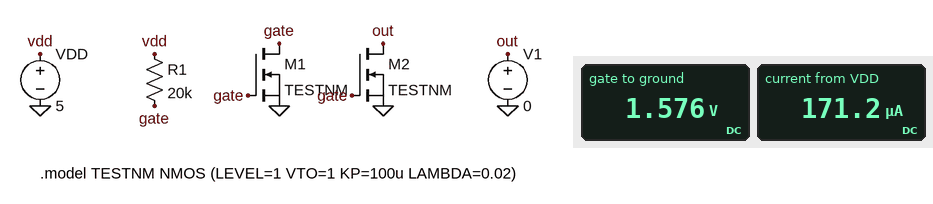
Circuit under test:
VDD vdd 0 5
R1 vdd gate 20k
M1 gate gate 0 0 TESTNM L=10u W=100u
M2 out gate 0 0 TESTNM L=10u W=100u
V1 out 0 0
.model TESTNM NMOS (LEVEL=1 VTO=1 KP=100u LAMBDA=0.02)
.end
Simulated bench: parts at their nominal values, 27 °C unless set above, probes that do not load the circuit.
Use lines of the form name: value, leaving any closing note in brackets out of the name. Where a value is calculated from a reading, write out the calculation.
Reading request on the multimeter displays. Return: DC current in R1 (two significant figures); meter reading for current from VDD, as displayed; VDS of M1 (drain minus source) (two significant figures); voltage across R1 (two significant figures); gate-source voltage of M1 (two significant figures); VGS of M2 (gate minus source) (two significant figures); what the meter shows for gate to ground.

DC current in R1: (5 V - 1.576 V) / 20 kΩ = 170 µA
meter reading for current from VDD, as displayed: 171.2 µA
VDS of M1 (drain minus source): 1.576 V = 1.6 V
voltage across R1: 5 V - 1.576 V = 3.4 V
gate-source voltage of M1: 1.576 V = 1.6 V
VGS of M2 (gate minus source): 1.576 V = 1.6 V
what the meter shows for gate to ground: 1.576 V
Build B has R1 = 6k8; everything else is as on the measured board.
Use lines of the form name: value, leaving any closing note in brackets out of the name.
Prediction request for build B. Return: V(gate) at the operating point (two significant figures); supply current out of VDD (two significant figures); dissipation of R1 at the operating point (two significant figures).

V(gate) at the operating point: 1.9 V
supply current out of VDD: 450 µA
dissipation of R1 at the operating point: 1.4 mW
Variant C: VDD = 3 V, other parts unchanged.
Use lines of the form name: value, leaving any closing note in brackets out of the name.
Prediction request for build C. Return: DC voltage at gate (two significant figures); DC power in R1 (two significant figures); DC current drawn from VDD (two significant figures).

DC voltage at gate: 1.4 V
DC power in R1: 130 µW
DC current drawn from VDD: 80 µA
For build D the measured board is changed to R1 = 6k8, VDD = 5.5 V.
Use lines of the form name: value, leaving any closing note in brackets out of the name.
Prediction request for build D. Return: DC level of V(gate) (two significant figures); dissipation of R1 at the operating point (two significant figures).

DC level of V(gate): 2.0 V
dissipation of R1 at the operating point: 1.8 mW
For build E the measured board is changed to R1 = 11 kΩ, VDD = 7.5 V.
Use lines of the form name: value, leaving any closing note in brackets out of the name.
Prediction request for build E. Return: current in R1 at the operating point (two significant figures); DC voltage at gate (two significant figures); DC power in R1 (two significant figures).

current in R1 at the operating point: 500 µA
DC voltage at gate: 2.0 V
DC power in R1: 2.8 mW
